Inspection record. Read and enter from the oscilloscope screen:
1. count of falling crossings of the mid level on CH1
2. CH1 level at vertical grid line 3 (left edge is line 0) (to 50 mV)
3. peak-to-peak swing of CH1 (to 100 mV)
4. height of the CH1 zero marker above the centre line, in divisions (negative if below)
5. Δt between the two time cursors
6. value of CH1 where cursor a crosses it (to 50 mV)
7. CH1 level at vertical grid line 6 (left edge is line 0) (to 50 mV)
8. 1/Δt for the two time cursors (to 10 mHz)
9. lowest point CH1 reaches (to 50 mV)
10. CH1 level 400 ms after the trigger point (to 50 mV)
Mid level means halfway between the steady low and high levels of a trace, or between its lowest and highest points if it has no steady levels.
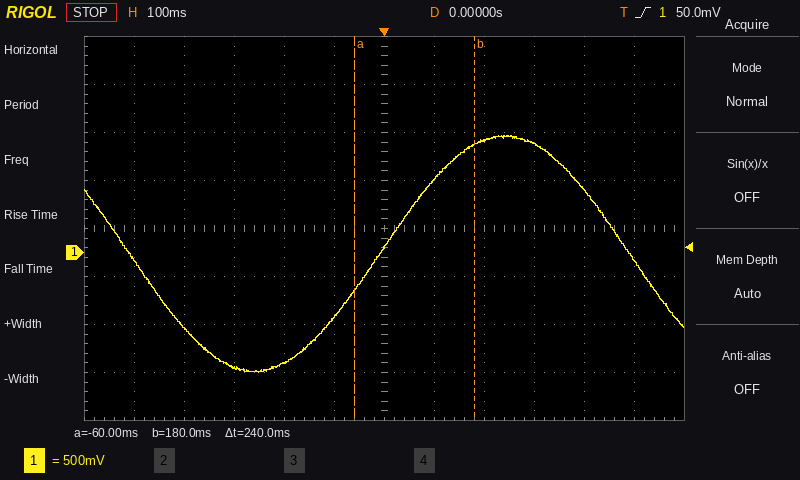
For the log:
2
-1.20 V
2.50 V
-0.5 div
240 ms
-400 mV
50 mV
4.17 Hz
-1.25 V
650 mV
